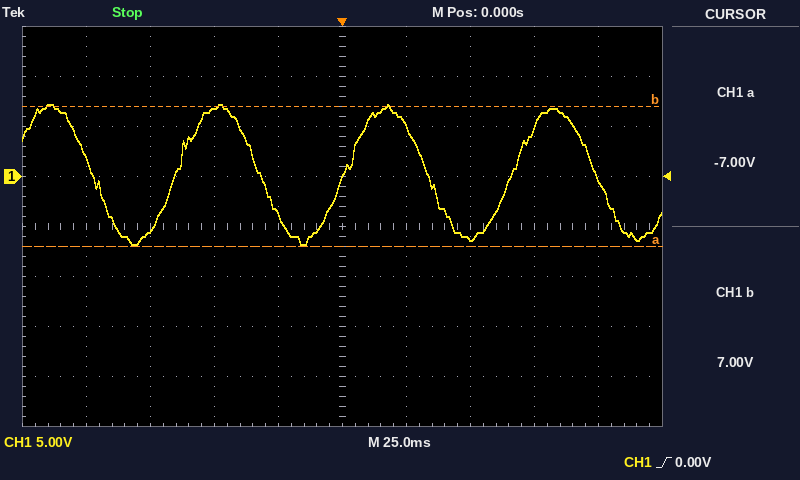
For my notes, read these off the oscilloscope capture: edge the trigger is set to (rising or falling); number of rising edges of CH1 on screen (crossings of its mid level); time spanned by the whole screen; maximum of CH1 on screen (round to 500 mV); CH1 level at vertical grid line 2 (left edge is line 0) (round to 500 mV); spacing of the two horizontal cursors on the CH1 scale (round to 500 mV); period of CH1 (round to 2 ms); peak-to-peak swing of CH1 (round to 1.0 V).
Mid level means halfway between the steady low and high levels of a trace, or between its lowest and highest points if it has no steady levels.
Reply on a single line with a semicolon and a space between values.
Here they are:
rising; 3; 250 ms; 7.0 V; -5.5 V; 14.0 V; 66 ms; 14.0 V
